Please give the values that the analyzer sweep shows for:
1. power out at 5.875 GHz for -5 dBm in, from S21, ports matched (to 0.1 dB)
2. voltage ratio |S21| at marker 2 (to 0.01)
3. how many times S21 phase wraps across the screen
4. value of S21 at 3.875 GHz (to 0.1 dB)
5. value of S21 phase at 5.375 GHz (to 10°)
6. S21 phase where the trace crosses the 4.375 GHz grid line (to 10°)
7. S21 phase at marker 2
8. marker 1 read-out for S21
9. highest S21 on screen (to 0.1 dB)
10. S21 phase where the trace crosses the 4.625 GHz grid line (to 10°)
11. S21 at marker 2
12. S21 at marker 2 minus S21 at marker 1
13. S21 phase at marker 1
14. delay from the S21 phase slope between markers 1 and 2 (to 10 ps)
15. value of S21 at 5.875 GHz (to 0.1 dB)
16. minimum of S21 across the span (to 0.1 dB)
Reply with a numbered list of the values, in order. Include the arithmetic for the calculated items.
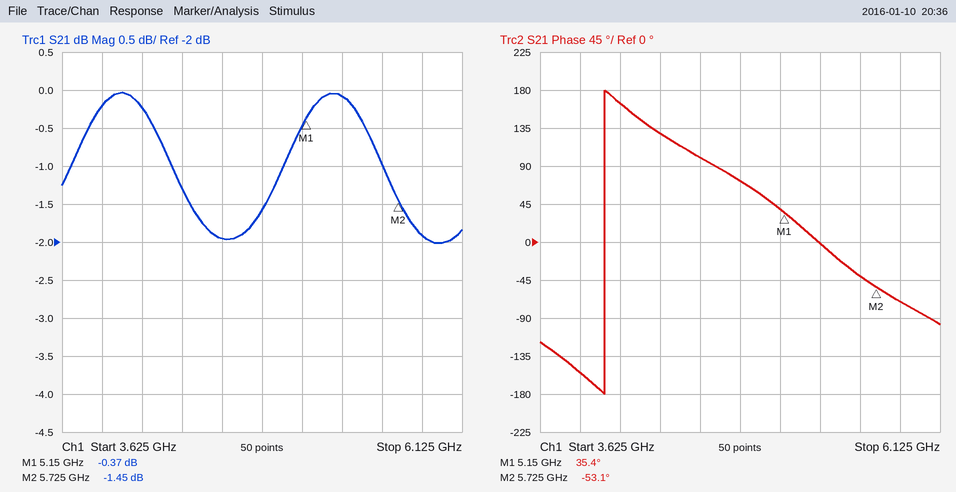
1. -5 dBm + (-1.9 dB) = -6.9 dBm
2. 10^(-1.45/20) ≈ 0.85
3. 1
4. -0.2 dB
5. 0°
6. 130°
7. -53.1°
8. -0.37 dB
9. 0.0 dB
10. 100°
11. -1.45 dB
12. -1.45 − (-0.37) = -1.08 dB
13. 35.4°
14. −(-53.1° − (35.4°))/(360° × 575 MHz) ≈ 428 ps, so 430 ps to the nearest 10 ps
15. -1.9 dB
16. -2.0 dB
